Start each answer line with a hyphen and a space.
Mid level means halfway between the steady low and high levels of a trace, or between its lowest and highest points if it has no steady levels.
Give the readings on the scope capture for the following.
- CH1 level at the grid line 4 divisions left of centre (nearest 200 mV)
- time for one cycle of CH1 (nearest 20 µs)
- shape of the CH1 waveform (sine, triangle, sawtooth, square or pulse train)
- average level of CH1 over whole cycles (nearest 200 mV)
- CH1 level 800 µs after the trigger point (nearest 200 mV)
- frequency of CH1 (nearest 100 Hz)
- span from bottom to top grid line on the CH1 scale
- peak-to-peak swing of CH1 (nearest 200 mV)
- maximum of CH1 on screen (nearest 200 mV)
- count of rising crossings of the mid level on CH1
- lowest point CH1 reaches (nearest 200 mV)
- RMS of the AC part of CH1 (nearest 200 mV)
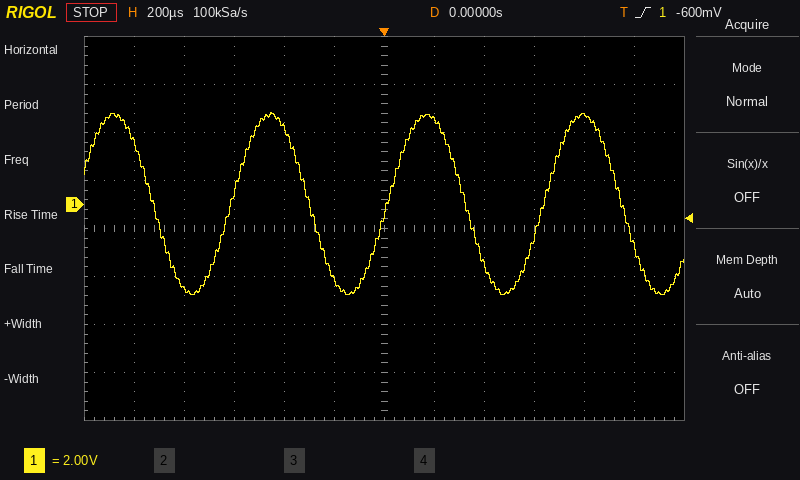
- -3.6 V
- 620 µs
- sine
- 0.0 V
- 3.8 V
- 1.6 kHz
- 16 V
- 7.6 V
- 3.8 V
- 3
- -3.8 V
- 2.6 V
